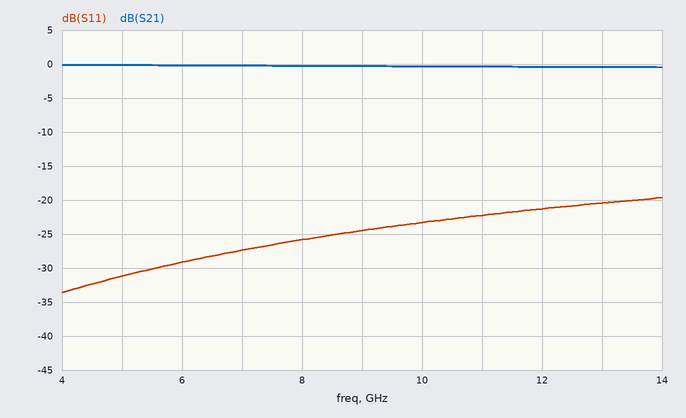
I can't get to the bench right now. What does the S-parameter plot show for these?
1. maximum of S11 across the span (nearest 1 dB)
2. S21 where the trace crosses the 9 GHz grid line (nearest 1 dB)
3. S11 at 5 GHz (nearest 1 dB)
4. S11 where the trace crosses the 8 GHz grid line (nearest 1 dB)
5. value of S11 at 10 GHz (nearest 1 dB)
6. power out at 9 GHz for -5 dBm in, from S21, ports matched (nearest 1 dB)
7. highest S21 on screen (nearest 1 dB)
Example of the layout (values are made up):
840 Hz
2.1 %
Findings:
-20 dB
0 dB
-31 dB
-26 dB
-23 dB
-5 dBm
0 dB
